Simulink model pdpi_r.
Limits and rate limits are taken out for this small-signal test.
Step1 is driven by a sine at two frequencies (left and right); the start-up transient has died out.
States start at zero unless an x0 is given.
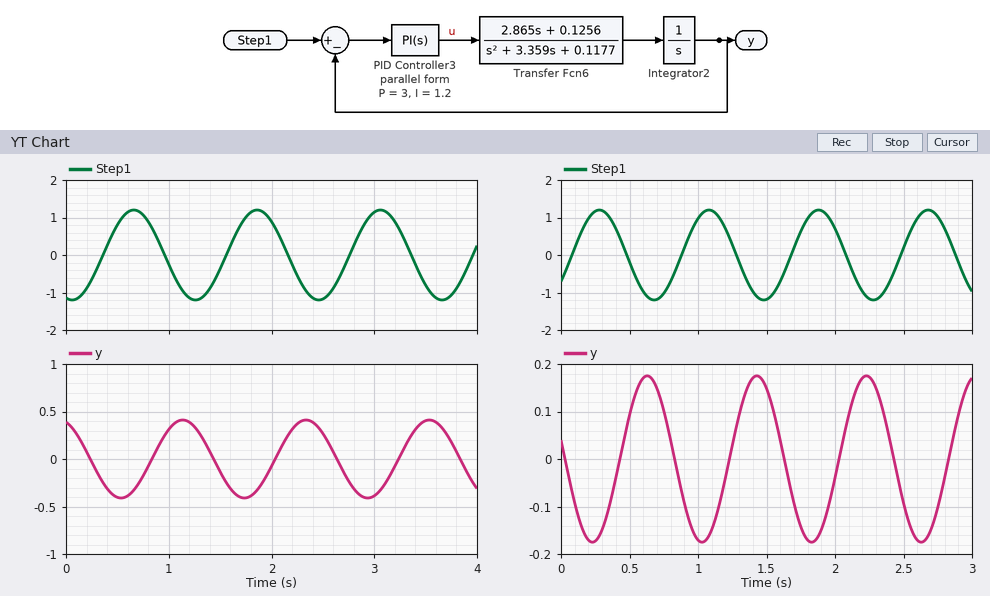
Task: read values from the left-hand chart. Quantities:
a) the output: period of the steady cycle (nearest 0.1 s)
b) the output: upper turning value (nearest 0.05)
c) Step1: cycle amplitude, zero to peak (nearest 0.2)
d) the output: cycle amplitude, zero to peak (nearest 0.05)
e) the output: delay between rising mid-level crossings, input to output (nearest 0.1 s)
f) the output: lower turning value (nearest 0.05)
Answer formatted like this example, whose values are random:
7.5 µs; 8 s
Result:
1.2 s; 0.40; 1.2; 0.40; 0.5 s; -0.40
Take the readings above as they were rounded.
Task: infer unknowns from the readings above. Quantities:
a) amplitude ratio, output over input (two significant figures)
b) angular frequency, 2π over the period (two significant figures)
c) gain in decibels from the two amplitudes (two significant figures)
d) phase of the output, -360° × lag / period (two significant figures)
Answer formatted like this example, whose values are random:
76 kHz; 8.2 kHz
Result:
0.33; 5.2 rad/s; -9.5 dB; -150°
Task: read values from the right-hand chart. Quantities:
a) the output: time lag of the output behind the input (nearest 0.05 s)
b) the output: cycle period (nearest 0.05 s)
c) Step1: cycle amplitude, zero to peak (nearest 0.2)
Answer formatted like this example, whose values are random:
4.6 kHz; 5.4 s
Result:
0.35 s; 0.80 s; 1.2
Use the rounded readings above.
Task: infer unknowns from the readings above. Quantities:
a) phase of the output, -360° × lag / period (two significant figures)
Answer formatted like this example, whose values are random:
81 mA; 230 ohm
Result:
-160°
